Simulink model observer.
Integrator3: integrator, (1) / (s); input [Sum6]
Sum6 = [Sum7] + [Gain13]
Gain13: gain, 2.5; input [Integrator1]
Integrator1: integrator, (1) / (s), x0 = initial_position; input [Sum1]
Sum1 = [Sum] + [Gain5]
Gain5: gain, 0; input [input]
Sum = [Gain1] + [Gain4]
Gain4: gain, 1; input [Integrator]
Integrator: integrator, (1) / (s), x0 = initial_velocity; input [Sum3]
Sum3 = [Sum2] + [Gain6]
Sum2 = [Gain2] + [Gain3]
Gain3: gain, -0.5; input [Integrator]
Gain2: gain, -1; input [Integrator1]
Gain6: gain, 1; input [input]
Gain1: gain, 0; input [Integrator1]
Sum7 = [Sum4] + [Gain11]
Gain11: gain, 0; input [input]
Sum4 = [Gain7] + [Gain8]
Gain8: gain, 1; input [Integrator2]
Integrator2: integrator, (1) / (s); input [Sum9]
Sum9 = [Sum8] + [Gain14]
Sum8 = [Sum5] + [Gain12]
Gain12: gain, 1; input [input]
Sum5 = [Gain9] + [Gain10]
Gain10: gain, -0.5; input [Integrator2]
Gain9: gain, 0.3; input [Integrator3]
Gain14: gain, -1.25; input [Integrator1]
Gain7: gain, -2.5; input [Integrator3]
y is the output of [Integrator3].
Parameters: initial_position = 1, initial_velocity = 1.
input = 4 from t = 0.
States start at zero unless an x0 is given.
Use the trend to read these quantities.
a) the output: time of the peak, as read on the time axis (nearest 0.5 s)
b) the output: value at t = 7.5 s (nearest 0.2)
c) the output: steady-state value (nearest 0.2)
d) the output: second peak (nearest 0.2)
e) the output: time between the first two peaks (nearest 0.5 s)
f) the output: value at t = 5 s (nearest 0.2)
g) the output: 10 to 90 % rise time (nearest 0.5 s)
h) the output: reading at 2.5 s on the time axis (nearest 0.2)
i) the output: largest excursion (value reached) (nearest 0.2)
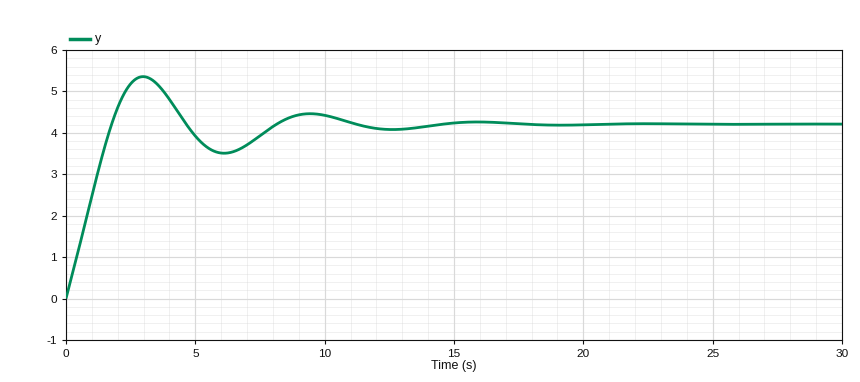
3.0 s
4.0
4.2
4.4
6.5 s
4.0
1.5 s
5.2
5.4
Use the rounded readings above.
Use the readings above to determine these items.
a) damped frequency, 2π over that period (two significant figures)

0.97 rad/s
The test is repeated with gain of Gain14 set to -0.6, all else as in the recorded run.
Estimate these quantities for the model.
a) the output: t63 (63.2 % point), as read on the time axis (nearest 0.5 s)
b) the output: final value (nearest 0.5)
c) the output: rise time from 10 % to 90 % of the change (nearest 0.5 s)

1.5 s
7.0
2.0 s
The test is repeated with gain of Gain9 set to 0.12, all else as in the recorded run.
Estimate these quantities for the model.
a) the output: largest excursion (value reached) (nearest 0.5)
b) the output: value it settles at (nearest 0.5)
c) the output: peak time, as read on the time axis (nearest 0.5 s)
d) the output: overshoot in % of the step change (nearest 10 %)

5.0
3.5
3.0 s
40 %
